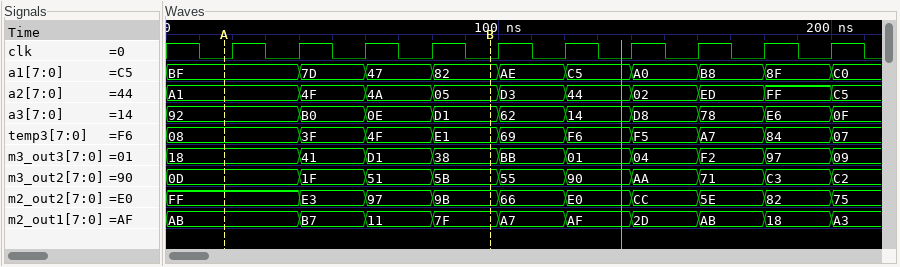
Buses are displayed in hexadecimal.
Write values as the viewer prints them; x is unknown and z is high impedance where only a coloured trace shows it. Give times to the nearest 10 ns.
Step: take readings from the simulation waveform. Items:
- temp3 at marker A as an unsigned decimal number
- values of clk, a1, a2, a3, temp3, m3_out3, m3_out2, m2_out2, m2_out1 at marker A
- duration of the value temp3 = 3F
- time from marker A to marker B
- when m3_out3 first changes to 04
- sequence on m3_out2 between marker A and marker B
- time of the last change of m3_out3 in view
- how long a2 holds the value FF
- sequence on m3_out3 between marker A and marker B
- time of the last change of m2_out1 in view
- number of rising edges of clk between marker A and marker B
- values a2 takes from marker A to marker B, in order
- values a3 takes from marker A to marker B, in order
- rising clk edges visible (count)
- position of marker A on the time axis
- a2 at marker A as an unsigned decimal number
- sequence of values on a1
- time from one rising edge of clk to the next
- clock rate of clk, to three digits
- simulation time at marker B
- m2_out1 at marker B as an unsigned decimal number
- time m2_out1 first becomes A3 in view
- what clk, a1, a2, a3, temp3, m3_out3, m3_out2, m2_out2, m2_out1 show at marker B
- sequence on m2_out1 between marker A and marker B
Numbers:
8
clk=0, a1=BF, a2=A1, a3=92, temp3=08, m3_out3=18, m3_out2=0D, m2_out2=FF, m2_out1=AB
20 ns
80 ns
140 ns
0D, 1F, 51, 5B
200 ns
20 ns
18, 41, D1, 38
200 ns
4
A1, 4F, 4A, 05
92, B0, 0E, D1
10
20 ns
161
BF, 7D, 47, 82, AE, C5, A0, B8, 8F, C0
20 ns
50.0 MHz
100 ns
127
200 ns
clk=0, a1=82, a2=05, a3=D1, temp3=E1, m3_out3=38, m3_out2=5B, m2_out2=9B, m2_out1=7F
AB, B7, 11, 7F
